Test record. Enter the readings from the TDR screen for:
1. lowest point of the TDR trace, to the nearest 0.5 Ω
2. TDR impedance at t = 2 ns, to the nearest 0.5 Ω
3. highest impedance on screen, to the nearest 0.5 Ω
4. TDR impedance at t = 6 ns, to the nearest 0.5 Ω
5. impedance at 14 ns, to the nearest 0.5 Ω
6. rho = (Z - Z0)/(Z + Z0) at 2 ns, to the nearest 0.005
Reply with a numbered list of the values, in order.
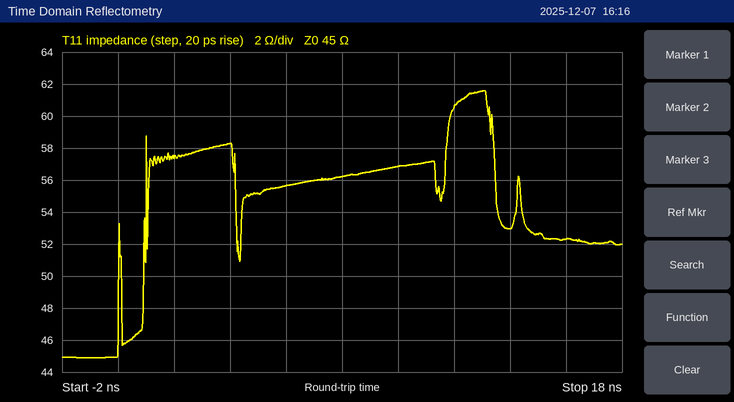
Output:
1. 45.0 Ω
2. 57.5 Ω
3. 61.5 Ω
4. 55.5 Ω
5. 53.0 Ω
6. +0.120
